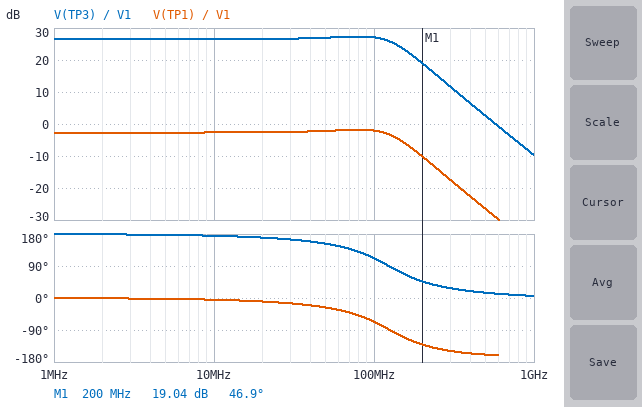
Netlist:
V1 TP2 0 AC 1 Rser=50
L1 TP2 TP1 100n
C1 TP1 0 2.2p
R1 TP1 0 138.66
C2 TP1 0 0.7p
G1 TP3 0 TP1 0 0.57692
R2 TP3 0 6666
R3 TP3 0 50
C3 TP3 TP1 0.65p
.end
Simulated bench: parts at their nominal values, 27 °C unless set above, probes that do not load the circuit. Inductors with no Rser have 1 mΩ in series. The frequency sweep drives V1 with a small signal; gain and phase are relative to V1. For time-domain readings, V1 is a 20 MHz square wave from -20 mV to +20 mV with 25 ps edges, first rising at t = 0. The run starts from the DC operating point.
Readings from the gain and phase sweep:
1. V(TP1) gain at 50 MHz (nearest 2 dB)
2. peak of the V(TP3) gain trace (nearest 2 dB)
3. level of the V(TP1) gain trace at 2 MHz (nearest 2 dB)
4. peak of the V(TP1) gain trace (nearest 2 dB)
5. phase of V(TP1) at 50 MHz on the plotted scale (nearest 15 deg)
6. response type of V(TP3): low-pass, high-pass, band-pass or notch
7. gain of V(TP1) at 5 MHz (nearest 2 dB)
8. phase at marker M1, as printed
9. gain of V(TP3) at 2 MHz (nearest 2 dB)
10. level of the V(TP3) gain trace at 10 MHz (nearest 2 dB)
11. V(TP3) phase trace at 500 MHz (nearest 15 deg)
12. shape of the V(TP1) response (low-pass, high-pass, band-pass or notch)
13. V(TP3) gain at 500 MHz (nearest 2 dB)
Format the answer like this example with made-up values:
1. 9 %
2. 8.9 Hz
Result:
1. -2 dB
2. 28 dB
3. -2 dB
4. -2 dB
5. -30 deg
6. low-pass
7. -2 dB
8. 46.9 deg
9. 26 dB
10. 26 dB
11. 15 deg
12. low-pass
13. 2 dB
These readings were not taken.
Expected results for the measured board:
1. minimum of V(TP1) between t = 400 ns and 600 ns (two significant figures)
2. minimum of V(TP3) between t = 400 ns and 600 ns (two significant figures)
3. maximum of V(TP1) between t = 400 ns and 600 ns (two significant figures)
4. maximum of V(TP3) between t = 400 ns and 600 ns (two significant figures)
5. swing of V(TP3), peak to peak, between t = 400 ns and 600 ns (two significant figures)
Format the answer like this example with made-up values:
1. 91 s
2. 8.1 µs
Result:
1. -19 mV
2. -540 mV
3. 19 mV
4. 540 mV
5. 1.1 V
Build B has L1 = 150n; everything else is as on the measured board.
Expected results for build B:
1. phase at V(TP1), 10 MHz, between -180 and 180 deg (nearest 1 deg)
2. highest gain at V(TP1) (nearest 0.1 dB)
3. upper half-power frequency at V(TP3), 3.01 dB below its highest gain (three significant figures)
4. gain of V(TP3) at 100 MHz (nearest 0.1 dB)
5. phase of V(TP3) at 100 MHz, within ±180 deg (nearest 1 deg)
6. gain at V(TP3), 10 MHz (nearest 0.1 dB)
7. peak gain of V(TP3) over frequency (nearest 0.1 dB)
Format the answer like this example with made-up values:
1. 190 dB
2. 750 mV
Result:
1. -6 deg
2. -1.7 dB
3. 118 MHz
4. 26.2 dB
5. 91 deg
6. 26.5 dB
7. 27.5 dB
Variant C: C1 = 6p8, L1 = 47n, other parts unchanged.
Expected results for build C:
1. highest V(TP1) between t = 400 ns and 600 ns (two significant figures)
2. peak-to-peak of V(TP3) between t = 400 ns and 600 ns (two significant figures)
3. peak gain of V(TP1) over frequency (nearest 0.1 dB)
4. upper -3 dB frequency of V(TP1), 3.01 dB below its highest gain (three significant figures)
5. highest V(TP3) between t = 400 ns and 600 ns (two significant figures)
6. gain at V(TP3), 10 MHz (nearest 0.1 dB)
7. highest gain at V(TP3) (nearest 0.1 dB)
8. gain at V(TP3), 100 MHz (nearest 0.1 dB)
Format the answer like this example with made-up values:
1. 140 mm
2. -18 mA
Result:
1. 17 mV
2. 960 mV
3. -2.6 dB
4. 176 MHz
5. 480 mV
6. 26.5 dB
7. 26.6 dB
8. 26.4 dB
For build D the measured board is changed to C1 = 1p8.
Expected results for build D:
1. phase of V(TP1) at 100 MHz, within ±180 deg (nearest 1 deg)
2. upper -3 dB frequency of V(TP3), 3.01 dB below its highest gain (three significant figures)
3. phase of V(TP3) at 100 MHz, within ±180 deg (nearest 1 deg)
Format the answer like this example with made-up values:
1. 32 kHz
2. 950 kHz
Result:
1. -66 deg
2. 145 MHz
3. 113 deg
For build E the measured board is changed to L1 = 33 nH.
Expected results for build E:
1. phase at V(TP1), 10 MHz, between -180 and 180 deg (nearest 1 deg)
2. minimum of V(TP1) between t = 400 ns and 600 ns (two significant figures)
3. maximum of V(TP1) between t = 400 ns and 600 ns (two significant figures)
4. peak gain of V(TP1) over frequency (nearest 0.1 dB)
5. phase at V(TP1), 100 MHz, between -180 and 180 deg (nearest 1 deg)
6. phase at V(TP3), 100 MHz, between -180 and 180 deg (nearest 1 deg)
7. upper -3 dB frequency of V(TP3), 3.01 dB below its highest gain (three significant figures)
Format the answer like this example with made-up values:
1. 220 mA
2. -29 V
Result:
1. -4 deg
2. -16 mV
3. 16 mV
4. -2.7 dB
5. -38 deg
6. 141 deg
7. 221 MHz
